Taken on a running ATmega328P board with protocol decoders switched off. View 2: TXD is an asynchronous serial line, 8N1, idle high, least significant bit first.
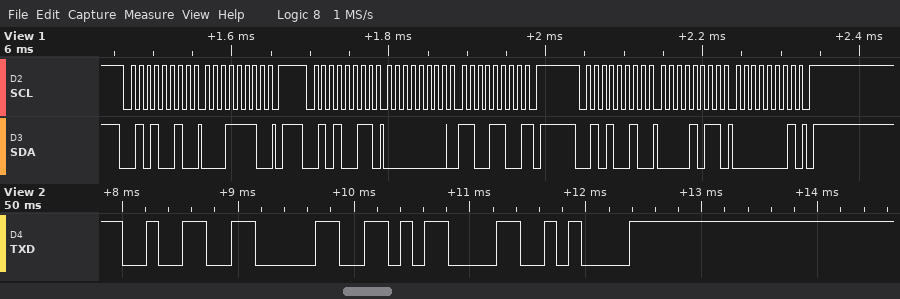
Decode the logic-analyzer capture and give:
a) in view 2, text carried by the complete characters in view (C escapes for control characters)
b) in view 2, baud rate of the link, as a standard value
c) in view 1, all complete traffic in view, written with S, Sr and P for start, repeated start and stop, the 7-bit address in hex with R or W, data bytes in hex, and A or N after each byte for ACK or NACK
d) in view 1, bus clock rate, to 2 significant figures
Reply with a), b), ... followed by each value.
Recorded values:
a) "20\r\n"
b) 9600 baud
c) S 29W A 1E A P S 29R A 00 A CC N P S 29W A 0B A 01 A P
d) 100 kHz
